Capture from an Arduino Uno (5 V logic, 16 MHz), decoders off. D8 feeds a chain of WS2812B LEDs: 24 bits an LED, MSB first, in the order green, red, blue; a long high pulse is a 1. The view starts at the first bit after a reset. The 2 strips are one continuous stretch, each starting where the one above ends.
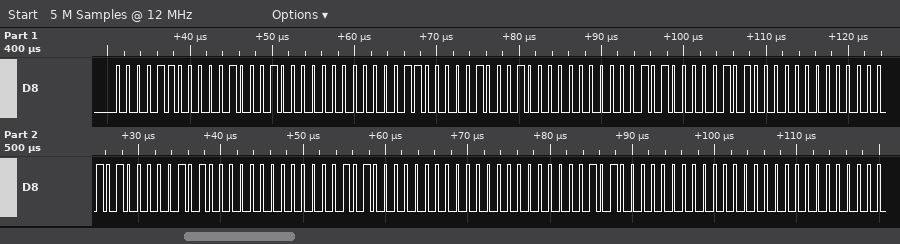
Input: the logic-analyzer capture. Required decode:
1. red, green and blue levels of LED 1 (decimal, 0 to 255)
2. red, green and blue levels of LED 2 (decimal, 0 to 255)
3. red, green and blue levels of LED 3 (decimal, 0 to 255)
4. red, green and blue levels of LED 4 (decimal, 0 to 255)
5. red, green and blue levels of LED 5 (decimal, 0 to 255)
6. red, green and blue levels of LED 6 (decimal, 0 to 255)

17, 12, 0
17, 12, 0
20, 20, 0
20, 20, 0
0, 20, 0
0, 20, 0
